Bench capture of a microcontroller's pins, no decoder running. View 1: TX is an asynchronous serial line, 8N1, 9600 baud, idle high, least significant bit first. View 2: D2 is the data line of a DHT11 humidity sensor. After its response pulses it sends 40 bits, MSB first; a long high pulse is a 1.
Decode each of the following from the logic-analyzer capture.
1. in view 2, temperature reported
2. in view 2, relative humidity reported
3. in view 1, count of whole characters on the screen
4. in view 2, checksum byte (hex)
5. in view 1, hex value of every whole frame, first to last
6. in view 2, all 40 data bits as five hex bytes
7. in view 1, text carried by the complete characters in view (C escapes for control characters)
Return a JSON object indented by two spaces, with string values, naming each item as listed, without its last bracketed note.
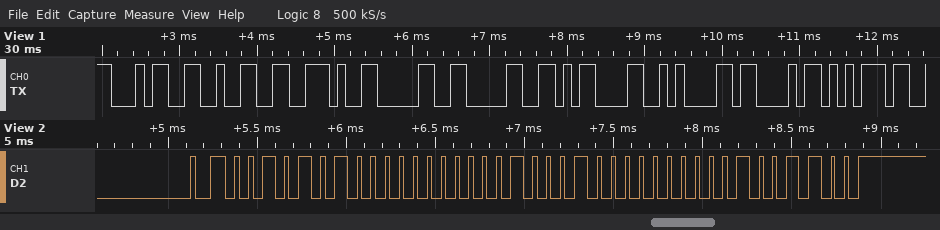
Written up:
{
  "in view 2, temperature reported": "34.0 °C",
  "in view 2, relative humidity reported": "42 %",
  "in view 1, count of whole characters on the screen": "9",
  "in view 2, checksum byte": "0x4C",
  "in view 1, hex value of every whole frame, first to last": "34 32 2E 30 30 0D 0A 43 75",
  "in view 2, all 40 data bits as five hex bytes": "2A 00 22 00 4C",
  "in view 1, text carried by the complete characters in view": "\"42.00\\r\\nCu\""
}
